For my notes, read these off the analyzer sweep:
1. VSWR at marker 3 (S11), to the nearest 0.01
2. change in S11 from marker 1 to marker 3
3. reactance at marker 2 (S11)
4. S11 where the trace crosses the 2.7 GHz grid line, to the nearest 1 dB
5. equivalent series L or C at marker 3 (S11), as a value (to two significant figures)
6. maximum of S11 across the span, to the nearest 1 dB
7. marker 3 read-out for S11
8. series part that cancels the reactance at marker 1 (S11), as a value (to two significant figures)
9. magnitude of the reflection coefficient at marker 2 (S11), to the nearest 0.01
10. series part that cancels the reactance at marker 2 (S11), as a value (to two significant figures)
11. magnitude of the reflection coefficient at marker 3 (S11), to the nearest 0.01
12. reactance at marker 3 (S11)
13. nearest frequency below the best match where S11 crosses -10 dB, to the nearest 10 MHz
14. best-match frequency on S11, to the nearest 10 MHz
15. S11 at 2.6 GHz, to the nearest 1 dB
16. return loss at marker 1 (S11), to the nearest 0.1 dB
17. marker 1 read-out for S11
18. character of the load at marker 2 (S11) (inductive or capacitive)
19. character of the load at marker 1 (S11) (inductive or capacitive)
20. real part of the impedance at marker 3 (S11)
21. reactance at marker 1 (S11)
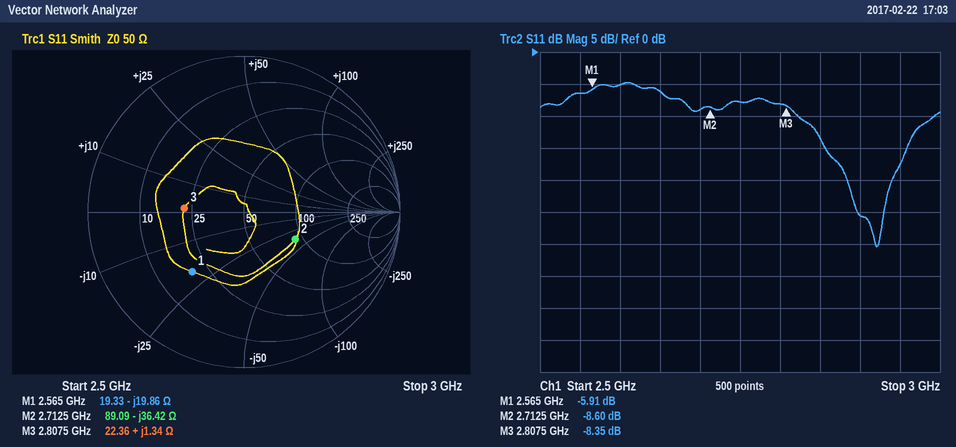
2.24
-2.44 dB
-36.42 Ω
-9 dB
76 pH
-5 dB
-8.35 dB
1.2 nH
0.37
2.1 nH
0.38
+1.34 Ω
2.82 GHz
2.92 GHz
-5 dB
5.9 dB
-5.91 dB
capacitive
capacitive
22.36 Ω
-19.86 Ω
